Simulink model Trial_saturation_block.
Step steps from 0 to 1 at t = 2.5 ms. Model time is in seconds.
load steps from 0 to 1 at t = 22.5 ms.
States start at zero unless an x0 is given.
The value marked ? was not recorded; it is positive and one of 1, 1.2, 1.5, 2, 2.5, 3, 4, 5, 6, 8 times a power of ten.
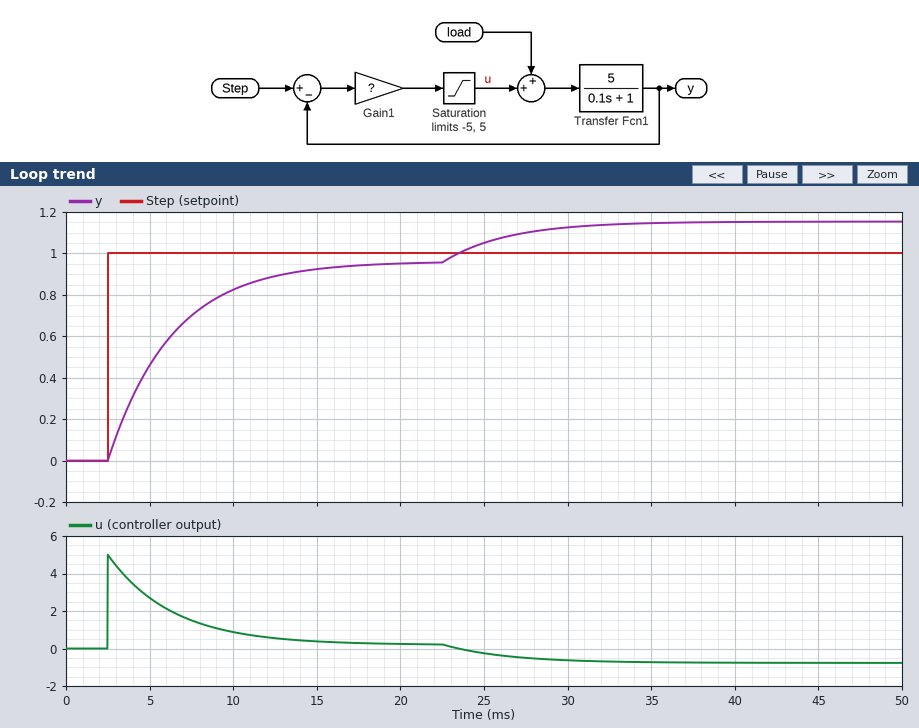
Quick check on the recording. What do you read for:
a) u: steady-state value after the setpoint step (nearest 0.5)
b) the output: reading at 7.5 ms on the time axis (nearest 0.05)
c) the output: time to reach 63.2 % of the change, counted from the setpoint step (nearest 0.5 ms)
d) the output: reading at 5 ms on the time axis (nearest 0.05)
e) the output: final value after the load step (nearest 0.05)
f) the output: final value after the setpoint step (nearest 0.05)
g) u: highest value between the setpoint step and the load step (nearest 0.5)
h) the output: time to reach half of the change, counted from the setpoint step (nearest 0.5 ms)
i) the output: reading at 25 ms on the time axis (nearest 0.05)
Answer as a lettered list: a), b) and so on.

a) 0.0
b) 0.70
c) 4.0 ms
d) 0.45
e) 1.15
f) 0.95
g) 5.0
h) 2.5 ms
i) 1.05
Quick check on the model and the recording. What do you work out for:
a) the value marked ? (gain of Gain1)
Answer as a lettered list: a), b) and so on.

a) 5
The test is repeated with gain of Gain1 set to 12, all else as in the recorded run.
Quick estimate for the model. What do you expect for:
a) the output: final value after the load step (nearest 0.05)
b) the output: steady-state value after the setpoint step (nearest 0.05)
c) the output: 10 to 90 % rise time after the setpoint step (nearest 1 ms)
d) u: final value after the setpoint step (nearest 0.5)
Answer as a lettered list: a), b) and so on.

a) 1.05
b) 1.00
c) 4 ms
d) 0.0
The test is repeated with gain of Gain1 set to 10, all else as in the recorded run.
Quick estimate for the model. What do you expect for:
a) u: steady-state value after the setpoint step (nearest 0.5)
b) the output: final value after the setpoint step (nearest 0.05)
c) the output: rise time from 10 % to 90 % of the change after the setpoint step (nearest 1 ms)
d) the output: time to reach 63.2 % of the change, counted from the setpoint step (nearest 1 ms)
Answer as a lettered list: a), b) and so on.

a) 0.0
b) 1.00
c) 5 ms
d) 3 ms
